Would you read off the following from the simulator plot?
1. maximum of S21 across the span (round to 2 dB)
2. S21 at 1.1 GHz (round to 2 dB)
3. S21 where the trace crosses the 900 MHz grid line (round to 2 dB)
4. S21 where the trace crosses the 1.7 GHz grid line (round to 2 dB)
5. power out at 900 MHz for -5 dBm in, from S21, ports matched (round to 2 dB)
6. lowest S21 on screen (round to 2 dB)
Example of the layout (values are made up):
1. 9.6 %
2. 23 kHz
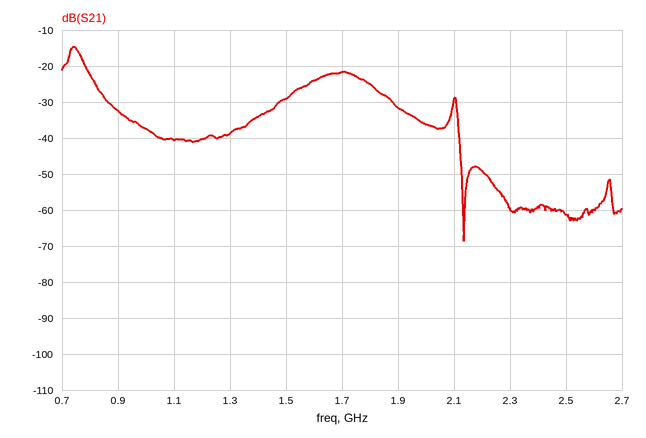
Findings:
1. -14 dB
2. -40 dB
3. -32 dB
4. -22 dB
5. -38 dBm
6. -68 dB
